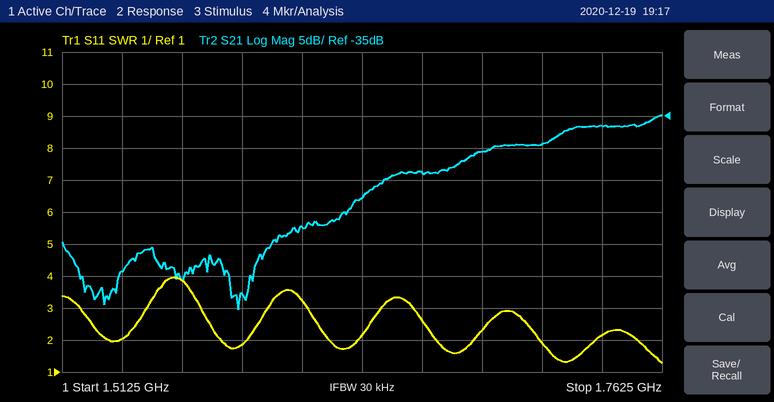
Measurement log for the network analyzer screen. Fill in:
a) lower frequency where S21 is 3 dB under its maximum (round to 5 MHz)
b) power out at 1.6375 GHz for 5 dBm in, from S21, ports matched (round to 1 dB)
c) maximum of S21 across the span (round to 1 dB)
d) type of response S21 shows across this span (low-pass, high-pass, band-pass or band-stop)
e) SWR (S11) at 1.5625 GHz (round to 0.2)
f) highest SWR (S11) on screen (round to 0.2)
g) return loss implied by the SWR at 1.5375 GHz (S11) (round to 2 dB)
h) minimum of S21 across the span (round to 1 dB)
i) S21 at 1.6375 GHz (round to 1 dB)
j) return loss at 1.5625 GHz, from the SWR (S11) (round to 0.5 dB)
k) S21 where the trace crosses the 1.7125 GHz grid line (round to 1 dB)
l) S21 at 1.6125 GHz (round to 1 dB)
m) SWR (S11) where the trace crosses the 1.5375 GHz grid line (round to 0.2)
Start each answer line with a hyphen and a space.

- 1.720 GHz
- -43 dBm
- -35 dB
- high-pass
- 3.8
- 4.0
- 10 dB
- -65 dB
- -48 dB
- 4.5 dB
- -39 dB
- -52 dB
- 2.0
